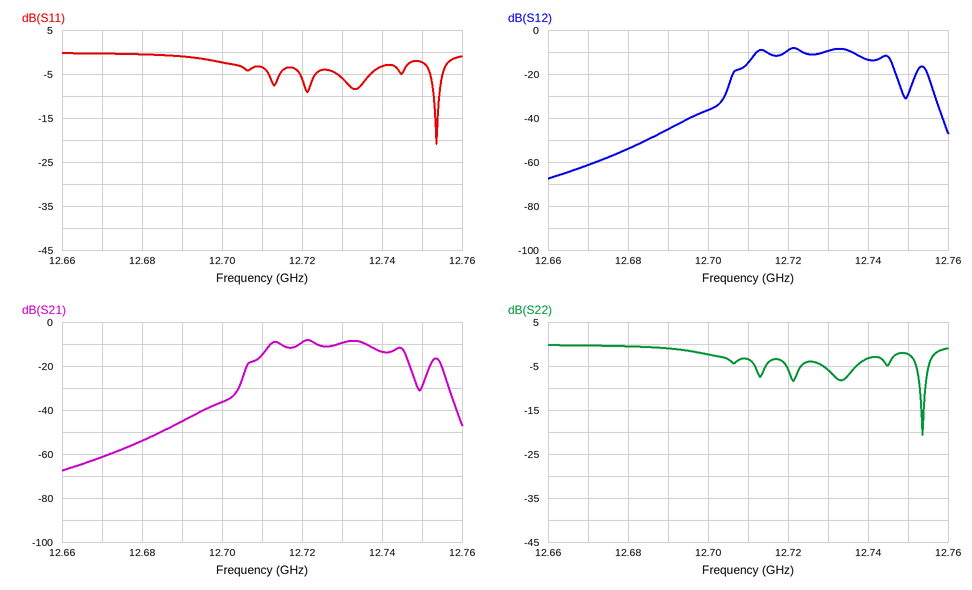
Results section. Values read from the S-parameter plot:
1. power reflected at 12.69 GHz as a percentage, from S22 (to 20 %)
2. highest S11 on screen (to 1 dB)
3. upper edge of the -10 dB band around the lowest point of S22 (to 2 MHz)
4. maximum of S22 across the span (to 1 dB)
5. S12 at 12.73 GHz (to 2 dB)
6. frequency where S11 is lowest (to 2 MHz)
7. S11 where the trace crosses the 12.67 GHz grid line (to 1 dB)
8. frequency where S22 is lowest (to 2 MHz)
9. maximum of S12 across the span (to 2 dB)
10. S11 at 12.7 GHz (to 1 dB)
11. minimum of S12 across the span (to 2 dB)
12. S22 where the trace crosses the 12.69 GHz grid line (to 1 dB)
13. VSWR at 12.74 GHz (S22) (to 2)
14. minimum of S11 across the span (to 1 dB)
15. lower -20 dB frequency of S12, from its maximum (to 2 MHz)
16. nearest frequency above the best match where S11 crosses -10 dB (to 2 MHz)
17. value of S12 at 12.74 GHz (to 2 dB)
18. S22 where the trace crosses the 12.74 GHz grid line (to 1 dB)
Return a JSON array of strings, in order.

["80 %", "0 dB", "12.754 GHz", "0 dB", "-10 dB", "12.754 GHz", "0 dB", "12.754 GHz", "-8 dB", "-2 dB", "-68 dB", "-1 dB", "6", "-21 dB", "12.704 GHz", "12.754 GHz", "-14 dB", "-3 dB"]
